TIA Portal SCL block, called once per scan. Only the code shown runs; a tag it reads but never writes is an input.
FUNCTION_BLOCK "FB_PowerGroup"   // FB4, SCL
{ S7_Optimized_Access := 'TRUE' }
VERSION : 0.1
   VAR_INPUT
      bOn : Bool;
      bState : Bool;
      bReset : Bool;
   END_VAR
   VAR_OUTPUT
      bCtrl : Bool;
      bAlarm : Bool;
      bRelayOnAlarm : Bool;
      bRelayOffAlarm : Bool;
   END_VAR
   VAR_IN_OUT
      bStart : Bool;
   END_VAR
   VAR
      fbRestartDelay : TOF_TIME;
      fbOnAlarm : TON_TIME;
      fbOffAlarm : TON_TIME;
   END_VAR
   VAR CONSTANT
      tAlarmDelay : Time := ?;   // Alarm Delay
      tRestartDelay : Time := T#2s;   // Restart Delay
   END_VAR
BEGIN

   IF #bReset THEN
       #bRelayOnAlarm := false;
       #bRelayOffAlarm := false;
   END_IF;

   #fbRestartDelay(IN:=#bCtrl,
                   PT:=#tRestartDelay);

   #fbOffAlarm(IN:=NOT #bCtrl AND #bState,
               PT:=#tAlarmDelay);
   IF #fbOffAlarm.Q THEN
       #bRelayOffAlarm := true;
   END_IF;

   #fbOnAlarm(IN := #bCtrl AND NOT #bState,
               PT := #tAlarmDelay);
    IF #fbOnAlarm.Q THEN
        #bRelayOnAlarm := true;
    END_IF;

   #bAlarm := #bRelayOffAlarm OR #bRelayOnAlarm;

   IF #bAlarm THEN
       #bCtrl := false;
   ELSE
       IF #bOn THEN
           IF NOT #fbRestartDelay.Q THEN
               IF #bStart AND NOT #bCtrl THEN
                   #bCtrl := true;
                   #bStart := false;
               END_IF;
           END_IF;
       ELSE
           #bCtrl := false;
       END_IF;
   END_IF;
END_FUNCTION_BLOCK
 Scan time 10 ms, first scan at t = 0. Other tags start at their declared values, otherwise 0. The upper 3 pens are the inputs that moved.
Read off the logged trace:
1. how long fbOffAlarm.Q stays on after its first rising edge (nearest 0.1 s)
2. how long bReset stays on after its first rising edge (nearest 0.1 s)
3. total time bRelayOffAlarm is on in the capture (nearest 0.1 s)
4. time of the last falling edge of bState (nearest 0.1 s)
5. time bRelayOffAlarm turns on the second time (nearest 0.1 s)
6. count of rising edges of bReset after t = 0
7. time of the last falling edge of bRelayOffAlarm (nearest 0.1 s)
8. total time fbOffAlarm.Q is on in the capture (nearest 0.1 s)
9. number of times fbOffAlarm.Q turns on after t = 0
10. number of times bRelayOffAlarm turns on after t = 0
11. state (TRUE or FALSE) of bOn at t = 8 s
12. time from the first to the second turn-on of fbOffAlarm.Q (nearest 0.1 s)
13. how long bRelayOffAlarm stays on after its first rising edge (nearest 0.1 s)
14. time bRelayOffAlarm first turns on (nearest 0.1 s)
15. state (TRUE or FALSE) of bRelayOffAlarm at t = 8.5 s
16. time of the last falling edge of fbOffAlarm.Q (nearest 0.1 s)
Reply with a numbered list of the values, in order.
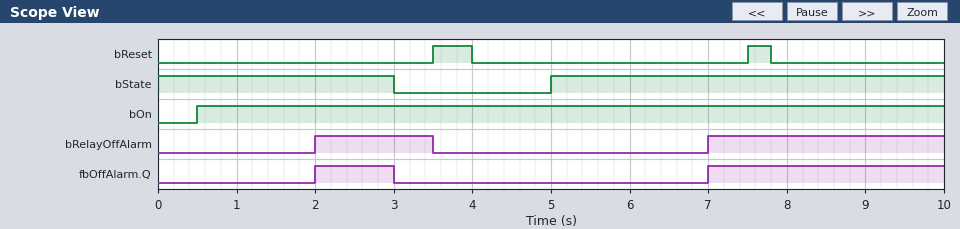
1. 1.0 s
2. 0.5 s
3. 4.5 s
4. 3.0 s
5. 7.0 s
6. 2
7. 3.5 s
8. 4.0 s
9. 2
10. 2
11. TRUE
12. 5.0 s
13. 1.5 s
14. 2.0 s
15. TRUE
16. 3.0 s
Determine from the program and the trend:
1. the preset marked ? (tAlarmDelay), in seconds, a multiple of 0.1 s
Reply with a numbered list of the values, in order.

1. 2.0 s
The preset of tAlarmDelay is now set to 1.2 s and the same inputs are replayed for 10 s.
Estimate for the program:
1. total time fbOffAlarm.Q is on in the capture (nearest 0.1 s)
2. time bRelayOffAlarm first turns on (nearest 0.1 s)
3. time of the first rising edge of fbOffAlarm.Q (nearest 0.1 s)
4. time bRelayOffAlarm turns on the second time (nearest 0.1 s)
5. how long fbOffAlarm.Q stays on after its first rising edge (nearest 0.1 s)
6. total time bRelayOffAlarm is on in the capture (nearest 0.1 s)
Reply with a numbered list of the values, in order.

1. 5.6 s
2. 1.2 s
3. 1.2 s
4. 6.2 s
5. 1.8 s
6. 6.1 s
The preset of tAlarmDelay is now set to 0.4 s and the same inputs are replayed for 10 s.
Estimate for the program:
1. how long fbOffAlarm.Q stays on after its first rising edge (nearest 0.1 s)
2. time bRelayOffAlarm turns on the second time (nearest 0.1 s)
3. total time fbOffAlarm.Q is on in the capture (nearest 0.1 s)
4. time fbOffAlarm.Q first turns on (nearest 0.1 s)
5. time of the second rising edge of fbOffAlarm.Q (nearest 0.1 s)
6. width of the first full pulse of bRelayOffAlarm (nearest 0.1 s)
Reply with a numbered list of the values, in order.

1. 2.6 s
2. 5.4 s
3. 7.2 s
4. 0.4 s
5. 5.4 s
6. 3.1 s
